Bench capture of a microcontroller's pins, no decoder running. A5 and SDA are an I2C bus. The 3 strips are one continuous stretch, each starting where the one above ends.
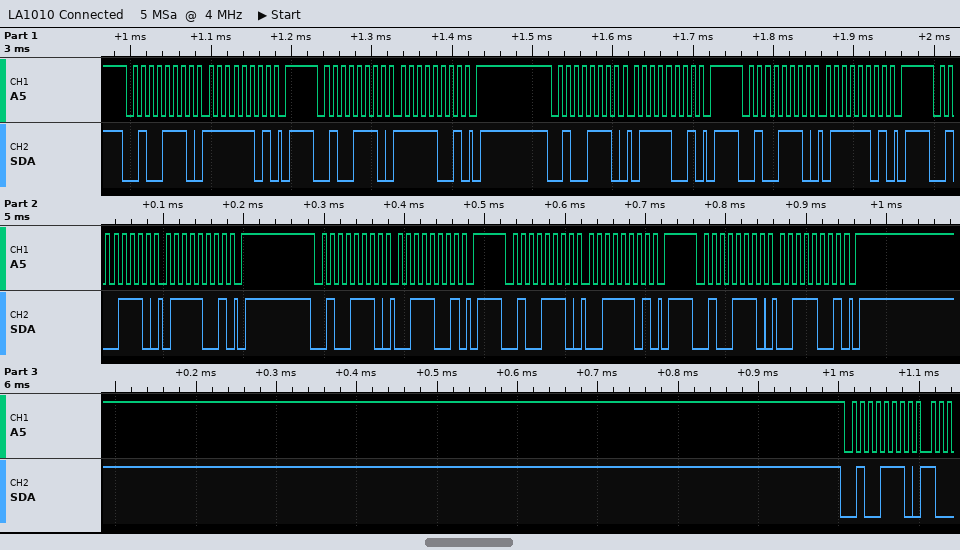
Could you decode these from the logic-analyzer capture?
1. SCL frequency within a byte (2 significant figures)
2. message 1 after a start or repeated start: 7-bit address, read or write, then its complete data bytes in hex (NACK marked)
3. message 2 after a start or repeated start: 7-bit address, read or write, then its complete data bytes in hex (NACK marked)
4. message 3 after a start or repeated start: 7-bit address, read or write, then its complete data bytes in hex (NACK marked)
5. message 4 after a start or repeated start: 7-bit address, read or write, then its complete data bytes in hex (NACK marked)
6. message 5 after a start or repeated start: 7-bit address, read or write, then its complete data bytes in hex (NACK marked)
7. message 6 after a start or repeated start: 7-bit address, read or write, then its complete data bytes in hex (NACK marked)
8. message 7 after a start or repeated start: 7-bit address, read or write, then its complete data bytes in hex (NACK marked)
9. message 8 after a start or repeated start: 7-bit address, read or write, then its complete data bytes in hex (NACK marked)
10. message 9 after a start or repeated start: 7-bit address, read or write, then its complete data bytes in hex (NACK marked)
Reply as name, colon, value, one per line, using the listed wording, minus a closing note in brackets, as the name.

SCL frequency within a byte: 100 kHz
message 1 after a start or repeated start: 7-bit address, read or write, then its complete data bytes in hex: 0x27 write: FD
message 2 after a start or repeated start: 7-bit address, read or write, then its complete data bytes in hex: 0x27 write: F9
message 3 after a start or repeated start: 7-bit address, read or write, then its complete data bytes in hex: 0x27 write: 79
message 4 after a start or repeated start: 7-bit address, read or write, then its complete data bytes in hex: 0x27 write: 7D
message 5 after a start or repeated start: 7-bit address, read or write, then its complete data bytes in hex: 0x27 write: 79
message 6 after a start or repeated start: 7-bit address, read or write, then its complete data bytes in hex: 0x27 write: 39
message 7 after a start or repeated start: 7-bit address, read or write, then its complete data bytes in hex: 0x27 write: 3D
message 8 after a start or repeated start: 7-bit address, read or write, then its complete data bytes in hex: 0x27 write: 39
message 9 after a start or repeated start: 7-bit address, read or write, then its complete data bytes in hex: 0x27 write
